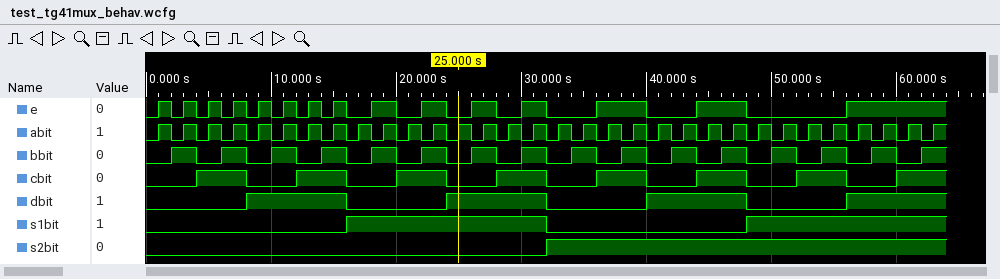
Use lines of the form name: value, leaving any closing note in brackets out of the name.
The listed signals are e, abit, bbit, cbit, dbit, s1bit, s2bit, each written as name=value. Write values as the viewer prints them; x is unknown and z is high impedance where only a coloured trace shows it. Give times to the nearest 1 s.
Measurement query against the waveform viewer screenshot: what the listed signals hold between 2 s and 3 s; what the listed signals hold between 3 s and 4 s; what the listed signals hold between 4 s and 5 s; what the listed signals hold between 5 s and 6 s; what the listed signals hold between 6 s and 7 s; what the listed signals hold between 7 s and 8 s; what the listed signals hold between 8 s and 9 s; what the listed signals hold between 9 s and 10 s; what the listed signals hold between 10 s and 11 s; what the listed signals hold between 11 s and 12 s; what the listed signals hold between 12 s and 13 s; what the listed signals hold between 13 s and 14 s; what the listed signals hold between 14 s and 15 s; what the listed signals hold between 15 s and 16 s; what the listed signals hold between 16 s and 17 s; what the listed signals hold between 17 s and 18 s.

what the listed signals hold between 2 s and 3 s: e=0, abit=0, bbit=1, cbit=0, dbit=0, s1bit=0, s2bit=0
what the listed signals hold between 3 s and 4 s: e=1, abit=1, bbit=1, cbit=0, dbit=0, s1bit=0, s2bit=0
what the listed signals hold between 4 s and 5 s: e=0, abit=0, bbit=0, cbit=1, dbit=0, s1bit=0, s2bit=0
what the listed signals hold between 5 s and 6 s: e=1, abit=1, bbit=0, cbit=1, dbit=0, s1bit=0, s2bit=0
what the listed signals hold between 6 s and 7 s: e=0, abit=0, bbit=1, cbit=1, dbit=0, s1bit=0, s2bit=0
what the listed signals hold between 7 s and 8 s: e=1, abit=1, bbit=1, cbit=1, dbit=0, s1bit=0, s2bit=0
what the listed signals hold between 8 s and 9 s: e=0, abit=0, bbit=0, cbit=0, dbit=1, s1bit=0, s2bit=0
what the listed signals hold between 9 s and 10 s: e=1, abit=1, bbit=0, cbit=0, dbit=1, s1bit=0, s2bit=0
what the listed signals hold between 10 s and 11 s: e=0, abit=0, bbit=1, cbit=0, dbit=1, s1bit=0, s2bit=0
what the listed signals hold between 11 s and 12 s: e=1, abit=1, bbit=1, cbit=0, dbit=1, s1bit=0, s2bit=0
what the listed signals hold between 12 s and 13 s: e=0, abit=0, bbit=0, cbit=1, dbit=1, s1bit=0, s2bit=0
what the listed signals hold between 13 s and 14 s: e=1, abit=1, bbit=0, cbit=1, dbit=1, s1bit=0, s2bit=0
what the listed signals hold between 14 s and 15 s: e=0, abit=0, bbit=1, cbit=1, dbit=1, s1bit=0, s2bit=0
what the listed signals hold between 15 s and 16 s: e=1, abit=1, bbit=1, cbit=1, dbit=1, s1bit=0, s2bit=0
what the listed signals hold between 16 s and 17 s: e=0, abit=0, bbit=0, cbit=0, dbit=0, s1bit=1, s2bit=0
what the listed signals hold between 17 s and 18 s: e=0, abit=1, bbit=0, cbit=0, dbit=0, s1bit=1, s2bit=0
